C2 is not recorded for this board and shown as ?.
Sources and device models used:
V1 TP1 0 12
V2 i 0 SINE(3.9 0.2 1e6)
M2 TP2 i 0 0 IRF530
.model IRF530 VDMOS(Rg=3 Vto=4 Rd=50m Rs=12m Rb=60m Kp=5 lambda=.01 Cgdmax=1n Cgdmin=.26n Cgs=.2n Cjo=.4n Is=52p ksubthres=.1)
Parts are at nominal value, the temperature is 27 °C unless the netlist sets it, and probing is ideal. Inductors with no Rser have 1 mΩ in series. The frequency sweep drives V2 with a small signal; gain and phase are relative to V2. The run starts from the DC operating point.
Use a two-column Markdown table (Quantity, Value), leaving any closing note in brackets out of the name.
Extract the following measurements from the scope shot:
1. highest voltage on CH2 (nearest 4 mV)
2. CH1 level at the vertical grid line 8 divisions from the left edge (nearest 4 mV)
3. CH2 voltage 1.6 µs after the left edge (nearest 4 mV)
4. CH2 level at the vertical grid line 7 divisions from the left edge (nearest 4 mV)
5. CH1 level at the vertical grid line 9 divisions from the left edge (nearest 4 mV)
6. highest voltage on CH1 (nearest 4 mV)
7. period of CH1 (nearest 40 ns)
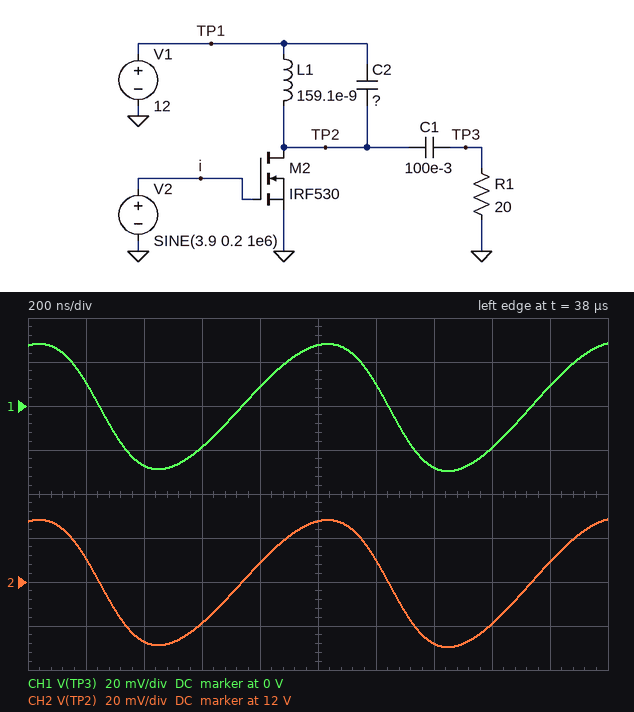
| Quantity | Value |
|---|---|
| highest voltage on CH2 | 12.028 V |
| CH1 level at the vertical grid line 8 divisions from the left edge | -20 mV |
| CH2 voltage 1.6 µs after the left edge | 11.980 V |
| CH2 level at the vertical grid line 7 divisions from the left edge | 11.972 V |
| CH1 level at the vertical grid line 9 divisions from the left edge | 8 mV |
| highest voltage on CH1 | 28 mV |
| period of CH1 | 1.00 µs |
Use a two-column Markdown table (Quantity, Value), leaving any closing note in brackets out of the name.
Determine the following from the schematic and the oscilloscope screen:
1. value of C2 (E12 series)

| Quantity | Value |
|---|---|
| value of C2 | 270 nF |
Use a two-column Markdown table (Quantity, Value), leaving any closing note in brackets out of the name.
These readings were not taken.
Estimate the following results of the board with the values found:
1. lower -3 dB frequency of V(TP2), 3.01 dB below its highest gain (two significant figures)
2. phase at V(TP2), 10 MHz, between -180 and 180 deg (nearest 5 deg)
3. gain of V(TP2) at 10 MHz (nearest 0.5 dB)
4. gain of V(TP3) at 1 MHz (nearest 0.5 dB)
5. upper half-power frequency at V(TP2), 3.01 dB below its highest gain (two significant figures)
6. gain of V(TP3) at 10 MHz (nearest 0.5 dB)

| Quantity | Value |
|---|---|
| lower -3 dB frequency of V(TP2), 3.01 dB below its highest gain | 750 kHz |
| phase at V(TP2), 10 MHz, between -180 and 180 deg | 65 deg |
| gain of V(TP2) at 10 MHz | -50.5 dB |
| gain of V(TP3) at 1 MHz | -23.5 dB |
| upper half-power frequency at V(TP2), 3.01 dB below its highest gain | 780 kHz |
| gain of V(TP3) at 10 MHz | -50.5 dB |
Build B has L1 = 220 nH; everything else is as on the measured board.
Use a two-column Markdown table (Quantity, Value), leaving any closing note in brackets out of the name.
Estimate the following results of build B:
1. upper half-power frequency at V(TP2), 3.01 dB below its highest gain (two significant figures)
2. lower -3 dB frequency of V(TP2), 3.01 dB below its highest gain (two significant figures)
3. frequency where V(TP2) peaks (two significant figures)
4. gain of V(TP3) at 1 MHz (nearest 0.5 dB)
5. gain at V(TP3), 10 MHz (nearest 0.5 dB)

| Quantity | Value |
|---|---|
| upper half-power frequency at V(TP2), 3.01 dB below its highest gain | 670 kHz |
| lower -3 dB frequency of V(TP2), 3.01 dB below its highest gain | 640 kHz |
| frequency where V(TP2) peaks | 650 kHz |
| gain of V(TP3) at 1 MHz | -26.5 dB |
| gain at V(TP3), 10 MHz | -50.5 dB |
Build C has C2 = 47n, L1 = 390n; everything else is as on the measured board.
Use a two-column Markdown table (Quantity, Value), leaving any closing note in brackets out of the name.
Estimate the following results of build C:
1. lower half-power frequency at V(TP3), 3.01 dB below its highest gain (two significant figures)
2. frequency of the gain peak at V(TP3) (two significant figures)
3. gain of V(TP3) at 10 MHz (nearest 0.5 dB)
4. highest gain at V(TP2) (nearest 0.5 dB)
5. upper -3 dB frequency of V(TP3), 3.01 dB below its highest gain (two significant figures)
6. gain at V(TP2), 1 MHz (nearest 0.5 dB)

| Quantity | Value |
|---|---|
| lower half-power frequency at V(TP3), 3.01 dB below its highest gain | 1.1 MHz |
| frequency of the gain peak at V(TP3) | 1.2 MHz |
| gain of V(TP3) at 10 MHz | -35.5 dB |
| highest gain at V(TP2) | -0.5 dB |
| upper -3 dB frequency of V(TP3), 3.01 dB below its highest gain | 1.3 MHz |
| gain at V(TP2), 1 MHz | -8.0 dB |
